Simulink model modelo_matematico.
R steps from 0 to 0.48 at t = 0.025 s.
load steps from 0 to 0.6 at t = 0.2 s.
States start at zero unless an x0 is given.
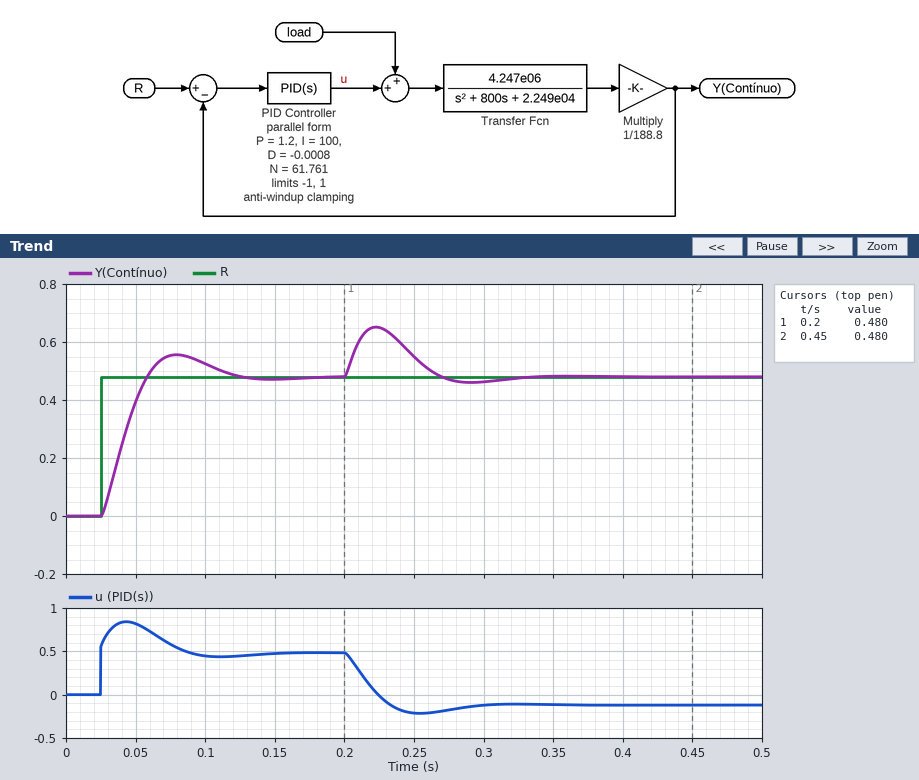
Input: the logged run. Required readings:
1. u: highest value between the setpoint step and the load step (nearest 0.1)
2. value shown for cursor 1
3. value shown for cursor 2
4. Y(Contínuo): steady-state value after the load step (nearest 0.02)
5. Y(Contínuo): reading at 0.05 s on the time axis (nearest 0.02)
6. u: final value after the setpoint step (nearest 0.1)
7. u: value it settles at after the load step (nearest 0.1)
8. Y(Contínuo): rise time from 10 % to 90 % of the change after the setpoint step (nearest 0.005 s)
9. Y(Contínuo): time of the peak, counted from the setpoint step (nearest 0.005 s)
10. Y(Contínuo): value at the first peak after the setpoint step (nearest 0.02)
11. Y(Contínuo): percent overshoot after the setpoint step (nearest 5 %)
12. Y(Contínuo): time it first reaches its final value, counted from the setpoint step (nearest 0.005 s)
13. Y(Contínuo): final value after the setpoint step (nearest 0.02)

0.8
0.480
0.480
0.48
0.40
0.5
-0.1
0.025 s
0.055 s
0.56
15 %
0.035 s
0.48
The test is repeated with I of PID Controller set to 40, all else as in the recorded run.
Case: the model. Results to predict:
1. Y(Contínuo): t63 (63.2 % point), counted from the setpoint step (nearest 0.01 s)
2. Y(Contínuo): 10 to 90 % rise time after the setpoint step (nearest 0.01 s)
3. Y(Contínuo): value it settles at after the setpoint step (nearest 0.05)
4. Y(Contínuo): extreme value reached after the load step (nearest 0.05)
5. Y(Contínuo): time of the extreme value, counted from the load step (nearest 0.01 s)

0.03 s
0.05 s
0.50
0.70
0.03 s
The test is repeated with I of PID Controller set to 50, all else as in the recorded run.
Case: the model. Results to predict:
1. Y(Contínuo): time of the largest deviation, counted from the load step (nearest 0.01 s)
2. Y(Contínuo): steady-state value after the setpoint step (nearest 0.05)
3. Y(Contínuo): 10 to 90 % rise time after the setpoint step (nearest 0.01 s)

0.03 s
0.50
0.04 s
